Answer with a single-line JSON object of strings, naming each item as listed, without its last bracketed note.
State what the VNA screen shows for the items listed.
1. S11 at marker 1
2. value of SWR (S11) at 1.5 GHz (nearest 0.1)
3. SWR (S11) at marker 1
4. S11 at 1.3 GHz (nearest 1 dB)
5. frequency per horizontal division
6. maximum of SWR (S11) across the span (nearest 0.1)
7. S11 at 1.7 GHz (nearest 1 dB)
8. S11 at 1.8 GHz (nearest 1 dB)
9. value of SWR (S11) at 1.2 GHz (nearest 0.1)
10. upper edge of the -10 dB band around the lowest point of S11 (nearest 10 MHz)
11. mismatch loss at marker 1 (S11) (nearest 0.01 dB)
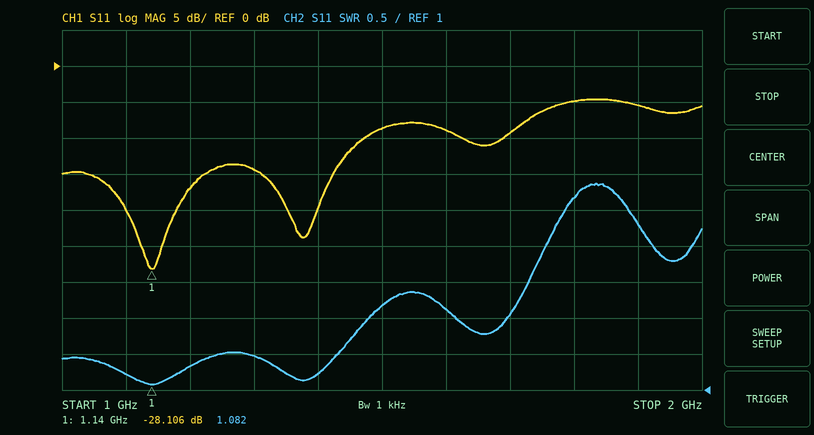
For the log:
{"S11 at marker 1": "-28.106 dB", "value of SWR (S11) at 1.5 GHz": "2.2", "SWR (S11) at marker 1": "1.082", "S11 at 1.3 GHz": "-14 dB", "frequency per horizontal division": "100 MHz", "maximum of SWR (S11) across the span": "3.9", "S11 at 1.7 GHz": "-9 dB", "S11 at 1.8 GHz": "-5 dB", "value of SWR (S11) at 1.2 GHz": "1.3", "upper edge of the -10 dB band around the lowest point of S11": "1.47 GHz", "mismatch loss at marker 1 (S11)": "0.01 dB"}
